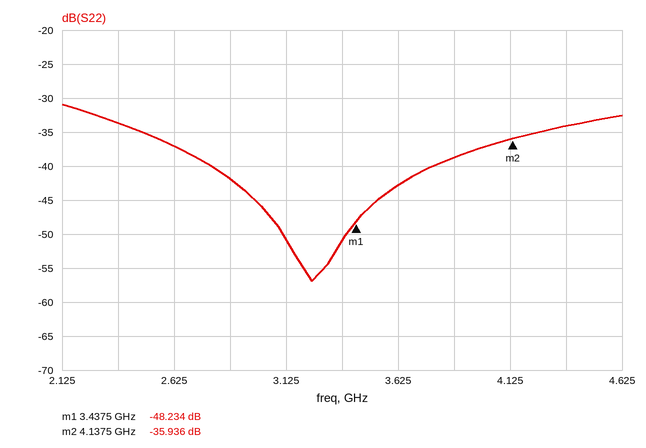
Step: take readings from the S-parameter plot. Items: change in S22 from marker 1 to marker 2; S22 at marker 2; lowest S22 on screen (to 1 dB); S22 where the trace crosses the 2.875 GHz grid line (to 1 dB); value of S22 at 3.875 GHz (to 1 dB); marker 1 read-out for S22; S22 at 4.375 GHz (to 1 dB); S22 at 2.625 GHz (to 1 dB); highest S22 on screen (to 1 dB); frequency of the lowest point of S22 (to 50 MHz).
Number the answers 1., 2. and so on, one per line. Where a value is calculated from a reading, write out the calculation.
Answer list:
1. -35.936 − (-48.234) = 12.298 dB
2. -35.936 dB
3. -57 dB
4. -42 dB
5. -39 dB
6. -48.234 dB
7. -34 dB
8. -37 dB
9. -31 dB
10. 3.25 GHz
